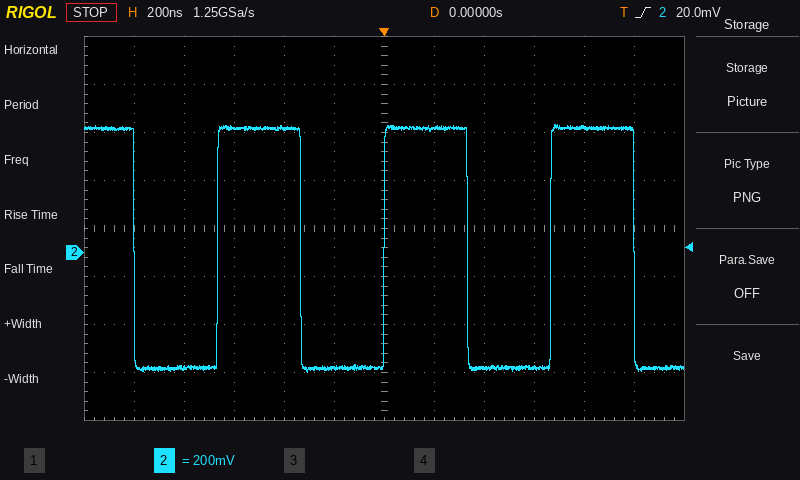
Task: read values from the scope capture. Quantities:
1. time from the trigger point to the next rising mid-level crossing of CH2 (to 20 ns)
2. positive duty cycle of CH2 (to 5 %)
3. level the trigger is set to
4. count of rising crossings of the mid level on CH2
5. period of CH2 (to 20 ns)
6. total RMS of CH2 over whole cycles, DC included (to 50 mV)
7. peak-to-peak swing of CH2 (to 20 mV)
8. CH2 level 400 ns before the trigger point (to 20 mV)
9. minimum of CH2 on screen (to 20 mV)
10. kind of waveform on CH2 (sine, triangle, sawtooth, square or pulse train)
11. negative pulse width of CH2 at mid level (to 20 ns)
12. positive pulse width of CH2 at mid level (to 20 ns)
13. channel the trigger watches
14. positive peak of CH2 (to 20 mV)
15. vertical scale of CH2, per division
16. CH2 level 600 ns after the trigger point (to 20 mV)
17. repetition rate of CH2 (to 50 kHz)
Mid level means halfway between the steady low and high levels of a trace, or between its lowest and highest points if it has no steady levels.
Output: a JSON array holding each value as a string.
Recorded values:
["660 ns", "50 %", "20.0 mV", "3", "660 ns", "500 mV", "1.04 V", "520 mV", "-500 mV", "square", "340 ns", "340 ns", "CH2", "540 mV", "200 mV", "-480 mV", "1.50 MHz"]
